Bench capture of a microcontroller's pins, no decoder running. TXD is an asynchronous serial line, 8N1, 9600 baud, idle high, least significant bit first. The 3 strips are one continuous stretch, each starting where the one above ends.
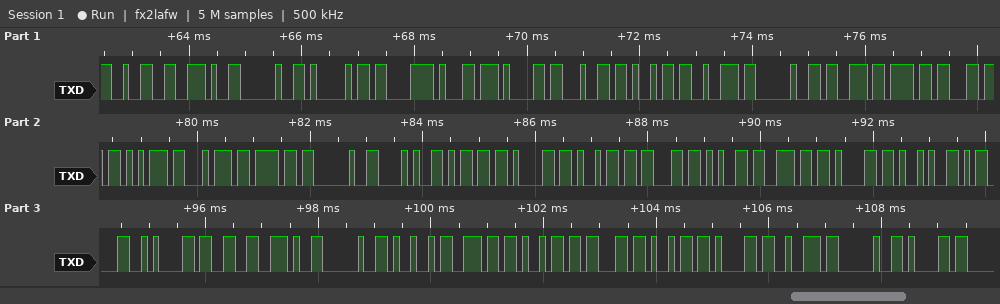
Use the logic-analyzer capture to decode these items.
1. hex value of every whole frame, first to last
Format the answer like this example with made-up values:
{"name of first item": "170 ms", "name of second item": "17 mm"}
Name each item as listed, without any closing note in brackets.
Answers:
{"hex value of every whole frame, first to last": "32 2E 20 41 C3 B1 61 64 69 72 20 73 6F 6C 75 74 6F 20 28 6D 61 69 63 65 6E 61 29 0D 0A 33 2E 20 49 6E 69 63 69 61 72 20 61"}
